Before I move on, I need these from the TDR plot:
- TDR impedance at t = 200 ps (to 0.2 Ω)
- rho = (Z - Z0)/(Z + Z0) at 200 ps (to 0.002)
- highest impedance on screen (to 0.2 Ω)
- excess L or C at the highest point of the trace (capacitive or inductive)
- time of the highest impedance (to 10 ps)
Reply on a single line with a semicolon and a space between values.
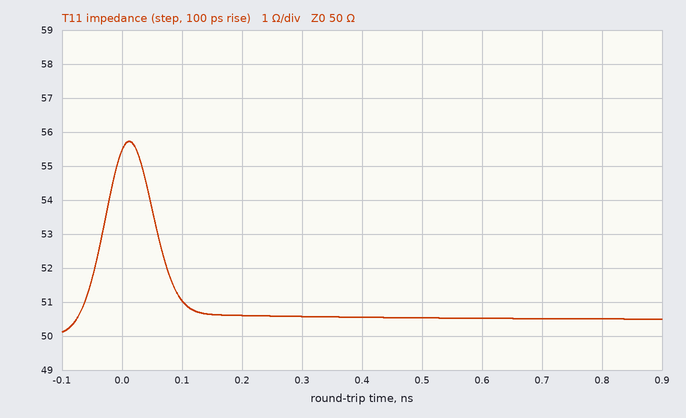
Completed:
50.6 Ω; +0.006; 55.8 Ω; inductive; 10 ps
